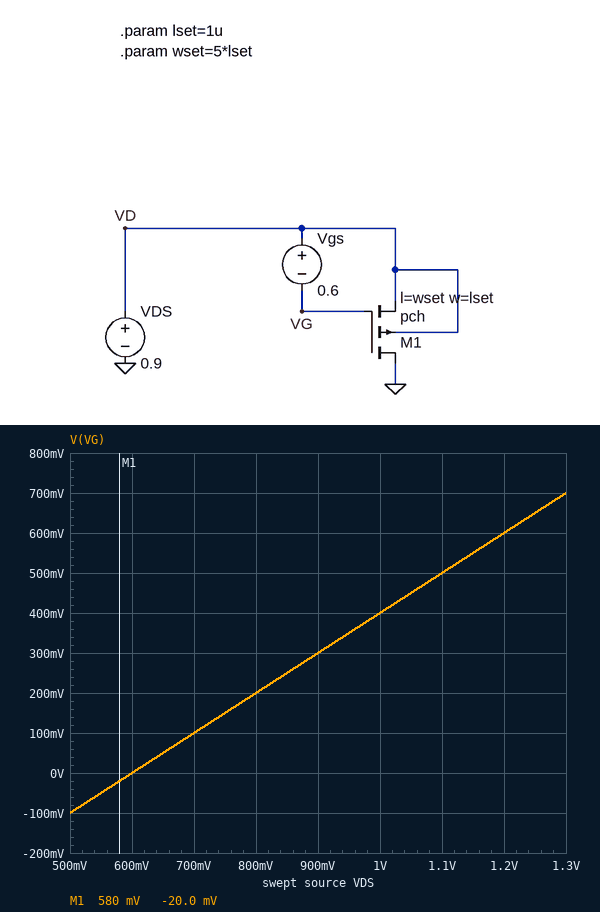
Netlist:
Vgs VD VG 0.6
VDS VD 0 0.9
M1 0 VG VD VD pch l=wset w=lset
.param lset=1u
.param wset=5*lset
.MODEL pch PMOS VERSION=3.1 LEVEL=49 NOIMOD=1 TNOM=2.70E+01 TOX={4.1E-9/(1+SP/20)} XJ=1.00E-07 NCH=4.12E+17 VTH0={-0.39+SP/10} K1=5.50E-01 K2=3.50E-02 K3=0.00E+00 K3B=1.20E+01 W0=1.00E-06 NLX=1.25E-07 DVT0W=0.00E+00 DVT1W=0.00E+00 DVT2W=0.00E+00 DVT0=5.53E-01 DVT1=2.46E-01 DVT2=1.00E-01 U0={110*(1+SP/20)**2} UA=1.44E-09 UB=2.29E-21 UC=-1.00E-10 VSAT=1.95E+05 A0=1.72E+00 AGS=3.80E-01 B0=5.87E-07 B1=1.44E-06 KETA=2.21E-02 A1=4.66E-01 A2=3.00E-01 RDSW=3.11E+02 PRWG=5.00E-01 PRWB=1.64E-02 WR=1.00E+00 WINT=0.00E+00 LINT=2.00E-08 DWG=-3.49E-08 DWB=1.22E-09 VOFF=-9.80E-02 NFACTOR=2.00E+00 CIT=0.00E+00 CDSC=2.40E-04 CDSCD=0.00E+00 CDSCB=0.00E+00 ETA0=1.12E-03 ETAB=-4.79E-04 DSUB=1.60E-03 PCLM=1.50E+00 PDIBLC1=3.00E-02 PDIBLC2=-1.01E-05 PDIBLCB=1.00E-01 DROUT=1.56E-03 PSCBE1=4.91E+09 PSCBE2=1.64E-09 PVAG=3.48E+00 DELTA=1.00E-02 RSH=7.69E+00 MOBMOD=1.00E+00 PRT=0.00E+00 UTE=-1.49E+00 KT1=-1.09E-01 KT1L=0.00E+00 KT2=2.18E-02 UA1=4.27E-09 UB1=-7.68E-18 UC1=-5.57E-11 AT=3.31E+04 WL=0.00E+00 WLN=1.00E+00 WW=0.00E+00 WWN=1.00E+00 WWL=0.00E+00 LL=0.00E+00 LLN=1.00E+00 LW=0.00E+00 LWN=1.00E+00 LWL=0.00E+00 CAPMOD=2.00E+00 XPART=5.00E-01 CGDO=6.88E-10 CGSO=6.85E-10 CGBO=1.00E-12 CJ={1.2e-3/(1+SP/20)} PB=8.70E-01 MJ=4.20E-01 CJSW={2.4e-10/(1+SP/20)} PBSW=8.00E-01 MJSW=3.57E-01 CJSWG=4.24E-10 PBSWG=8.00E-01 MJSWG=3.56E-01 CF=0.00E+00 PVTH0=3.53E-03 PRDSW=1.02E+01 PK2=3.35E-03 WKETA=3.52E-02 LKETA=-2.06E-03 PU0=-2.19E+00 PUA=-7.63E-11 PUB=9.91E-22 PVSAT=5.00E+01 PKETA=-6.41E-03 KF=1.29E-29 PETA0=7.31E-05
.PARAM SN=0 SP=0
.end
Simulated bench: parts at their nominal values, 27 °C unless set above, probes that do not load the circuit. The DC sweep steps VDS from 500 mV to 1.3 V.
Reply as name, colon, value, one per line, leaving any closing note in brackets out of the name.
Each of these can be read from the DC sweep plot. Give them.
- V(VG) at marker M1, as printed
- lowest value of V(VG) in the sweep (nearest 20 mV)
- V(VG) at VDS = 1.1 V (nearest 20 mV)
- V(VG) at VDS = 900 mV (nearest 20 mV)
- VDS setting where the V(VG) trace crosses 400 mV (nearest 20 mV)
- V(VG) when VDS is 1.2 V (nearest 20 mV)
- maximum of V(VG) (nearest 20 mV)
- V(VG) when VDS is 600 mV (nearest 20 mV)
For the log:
V(VG) at marker M1, as printed: -20.0 mV
lowest value of V(VG) in the sweep: -100 mV
V(VG) at VDS = 1.1 V: 500 mV
V(VG) at VDS = 900 mV: 300 mV
VDS setting where the V(VG) trace crosses 400 mV: 1.00 V
V(VG) when VDS is 1.2 V: 600 mV
maximum of V(VG): 700 mV
V(VG) when VDS is 600 mV: 0 V
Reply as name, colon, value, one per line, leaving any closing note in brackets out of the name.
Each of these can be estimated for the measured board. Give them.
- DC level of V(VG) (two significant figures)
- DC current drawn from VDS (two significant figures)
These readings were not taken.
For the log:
DC level of V(VG): 300 mV
DC current drawn from VDS: 230 nA
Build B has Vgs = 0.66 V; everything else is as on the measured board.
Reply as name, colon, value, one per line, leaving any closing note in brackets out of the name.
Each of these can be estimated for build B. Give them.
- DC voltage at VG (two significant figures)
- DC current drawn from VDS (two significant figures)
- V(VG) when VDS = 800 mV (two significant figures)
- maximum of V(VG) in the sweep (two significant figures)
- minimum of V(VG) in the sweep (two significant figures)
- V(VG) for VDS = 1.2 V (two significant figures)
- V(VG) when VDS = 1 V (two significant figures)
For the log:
DC voltage at VG: 240 mV
DC current drawn from VDS: 380 nA
V(VG) when VDS = 800 mV: 140 mV
maximum of V(VG) in the sweep: 640 mV
minimum of V(VG) in the sweep: -160 mV
V(VG) for VDS = 1.2 V: 540 mV
V(VG) when VDS = 1 V: 340 mV
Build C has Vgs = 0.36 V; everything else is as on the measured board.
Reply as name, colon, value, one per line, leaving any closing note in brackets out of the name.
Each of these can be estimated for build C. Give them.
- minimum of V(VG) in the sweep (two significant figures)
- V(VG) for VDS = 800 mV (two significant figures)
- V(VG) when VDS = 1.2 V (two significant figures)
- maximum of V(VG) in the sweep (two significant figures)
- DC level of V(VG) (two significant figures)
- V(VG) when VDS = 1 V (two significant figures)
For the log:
minimum of V(VG) in the sweep: 140 mV
V(VG) for VDS = 800 mV: 440 mV
V(VG) when VDS = 1.2 V: 840 mV
maximum of V(VG) in the sweep: 940 mV
DC level of V(VG): 540 mV
V(VG) when VDS = 1 V: 640 mV
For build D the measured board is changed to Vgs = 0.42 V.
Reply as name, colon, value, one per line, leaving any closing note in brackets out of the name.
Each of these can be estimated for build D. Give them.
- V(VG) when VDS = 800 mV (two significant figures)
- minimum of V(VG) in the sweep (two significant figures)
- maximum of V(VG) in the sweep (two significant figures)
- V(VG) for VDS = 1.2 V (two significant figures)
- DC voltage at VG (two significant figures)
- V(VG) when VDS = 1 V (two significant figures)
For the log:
V(VG) when VDS = 800 mV: 380 mV
minimum of V(VG) in the sweep: 80 mV
maximum of V(VG) in the sweep: 880 mV
V(VG) for VDS = 1.2 V: 780 mV
DC voltage at VG: 480 mV
V(VG) when VDS = 1 V: 580 mV
